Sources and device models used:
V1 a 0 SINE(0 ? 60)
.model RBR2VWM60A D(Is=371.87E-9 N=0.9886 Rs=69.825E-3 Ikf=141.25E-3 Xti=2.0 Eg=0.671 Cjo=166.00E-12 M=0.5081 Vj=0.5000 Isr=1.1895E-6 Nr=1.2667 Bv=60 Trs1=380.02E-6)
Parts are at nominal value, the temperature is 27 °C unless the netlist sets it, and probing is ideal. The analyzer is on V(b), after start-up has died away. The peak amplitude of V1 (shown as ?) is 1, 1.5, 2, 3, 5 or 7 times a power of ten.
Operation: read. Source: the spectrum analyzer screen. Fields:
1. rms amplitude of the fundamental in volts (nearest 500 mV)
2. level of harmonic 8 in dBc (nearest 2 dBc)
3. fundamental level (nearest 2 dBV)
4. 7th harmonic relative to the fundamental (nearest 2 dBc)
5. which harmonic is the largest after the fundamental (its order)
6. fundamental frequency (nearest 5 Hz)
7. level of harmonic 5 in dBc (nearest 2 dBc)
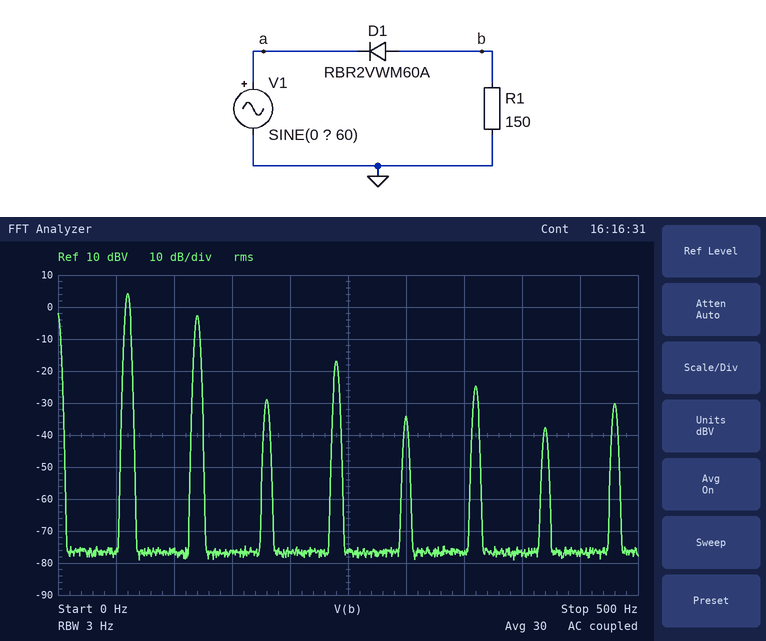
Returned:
1.5 V
-34 dBc
4 dBV
-42 dBc
2
60 Hz
-38 dBc
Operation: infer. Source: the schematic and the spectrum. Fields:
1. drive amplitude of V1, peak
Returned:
5 V
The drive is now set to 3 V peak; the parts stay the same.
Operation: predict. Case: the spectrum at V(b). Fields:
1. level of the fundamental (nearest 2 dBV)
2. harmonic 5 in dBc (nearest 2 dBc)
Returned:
0 dBV
-34 dBc
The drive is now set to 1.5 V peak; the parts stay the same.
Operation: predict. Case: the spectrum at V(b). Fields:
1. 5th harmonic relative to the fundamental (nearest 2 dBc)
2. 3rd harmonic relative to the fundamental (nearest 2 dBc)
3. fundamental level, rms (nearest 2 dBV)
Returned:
-30 dBc
-24 dBc
-8 dBV
